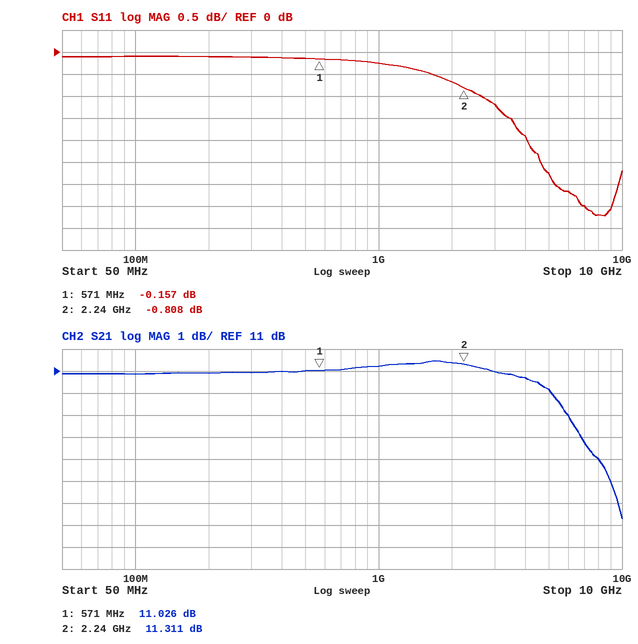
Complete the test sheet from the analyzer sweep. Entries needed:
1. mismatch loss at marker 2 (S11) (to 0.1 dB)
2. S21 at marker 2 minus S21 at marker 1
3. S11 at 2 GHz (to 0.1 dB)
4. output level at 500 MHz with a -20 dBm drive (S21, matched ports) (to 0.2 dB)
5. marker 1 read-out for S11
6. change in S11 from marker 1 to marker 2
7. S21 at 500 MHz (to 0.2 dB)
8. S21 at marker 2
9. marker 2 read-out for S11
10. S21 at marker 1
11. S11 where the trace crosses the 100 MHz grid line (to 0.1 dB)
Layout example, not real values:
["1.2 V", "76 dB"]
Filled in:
["7.7 dB", "0.285 dB", "-0.7 dB", "-9.0 dBm", "-0.157 dB", "-0.651 dB", "11.0 dB", "11.311 dB", "-0.808 dB", "11.026 dB", "-0.1 dB"]
